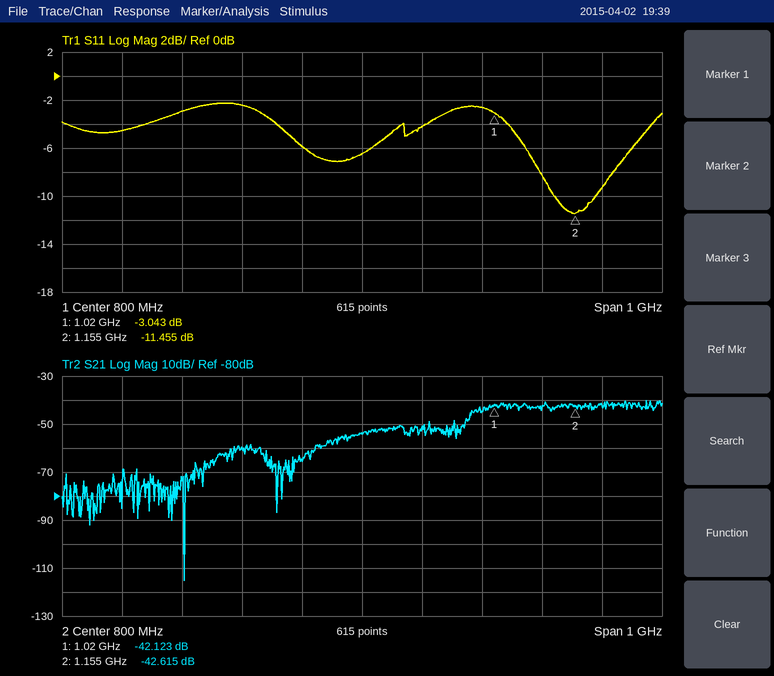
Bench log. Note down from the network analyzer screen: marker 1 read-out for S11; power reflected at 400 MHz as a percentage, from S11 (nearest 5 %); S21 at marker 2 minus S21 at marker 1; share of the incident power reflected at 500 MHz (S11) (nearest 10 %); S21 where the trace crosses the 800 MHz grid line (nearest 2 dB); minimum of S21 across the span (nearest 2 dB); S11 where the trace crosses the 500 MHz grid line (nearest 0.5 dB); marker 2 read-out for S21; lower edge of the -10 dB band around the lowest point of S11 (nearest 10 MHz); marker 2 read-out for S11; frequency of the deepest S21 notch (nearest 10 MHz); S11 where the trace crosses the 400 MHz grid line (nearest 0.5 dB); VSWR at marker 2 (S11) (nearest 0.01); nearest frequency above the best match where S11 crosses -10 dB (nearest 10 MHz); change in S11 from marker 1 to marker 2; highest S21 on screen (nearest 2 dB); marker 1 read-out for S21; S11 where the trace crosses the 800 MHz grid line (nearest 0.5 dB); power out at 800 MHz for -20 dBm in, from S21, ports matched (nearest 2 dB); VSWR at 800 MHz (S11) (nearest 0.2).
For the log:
-3.043 dB
35 %
-0.492 dB
50 %
-54 dB
-116 dB
-3.0 dB
-42.615 dB
1.12 GHz
-11.455 dB
500 MHz
-4.5 dB
1.73
1.19 GHz
-8.412 dB
-40 dB
-42.123 dB
-6.5 dB
-74 dBm
2.8
